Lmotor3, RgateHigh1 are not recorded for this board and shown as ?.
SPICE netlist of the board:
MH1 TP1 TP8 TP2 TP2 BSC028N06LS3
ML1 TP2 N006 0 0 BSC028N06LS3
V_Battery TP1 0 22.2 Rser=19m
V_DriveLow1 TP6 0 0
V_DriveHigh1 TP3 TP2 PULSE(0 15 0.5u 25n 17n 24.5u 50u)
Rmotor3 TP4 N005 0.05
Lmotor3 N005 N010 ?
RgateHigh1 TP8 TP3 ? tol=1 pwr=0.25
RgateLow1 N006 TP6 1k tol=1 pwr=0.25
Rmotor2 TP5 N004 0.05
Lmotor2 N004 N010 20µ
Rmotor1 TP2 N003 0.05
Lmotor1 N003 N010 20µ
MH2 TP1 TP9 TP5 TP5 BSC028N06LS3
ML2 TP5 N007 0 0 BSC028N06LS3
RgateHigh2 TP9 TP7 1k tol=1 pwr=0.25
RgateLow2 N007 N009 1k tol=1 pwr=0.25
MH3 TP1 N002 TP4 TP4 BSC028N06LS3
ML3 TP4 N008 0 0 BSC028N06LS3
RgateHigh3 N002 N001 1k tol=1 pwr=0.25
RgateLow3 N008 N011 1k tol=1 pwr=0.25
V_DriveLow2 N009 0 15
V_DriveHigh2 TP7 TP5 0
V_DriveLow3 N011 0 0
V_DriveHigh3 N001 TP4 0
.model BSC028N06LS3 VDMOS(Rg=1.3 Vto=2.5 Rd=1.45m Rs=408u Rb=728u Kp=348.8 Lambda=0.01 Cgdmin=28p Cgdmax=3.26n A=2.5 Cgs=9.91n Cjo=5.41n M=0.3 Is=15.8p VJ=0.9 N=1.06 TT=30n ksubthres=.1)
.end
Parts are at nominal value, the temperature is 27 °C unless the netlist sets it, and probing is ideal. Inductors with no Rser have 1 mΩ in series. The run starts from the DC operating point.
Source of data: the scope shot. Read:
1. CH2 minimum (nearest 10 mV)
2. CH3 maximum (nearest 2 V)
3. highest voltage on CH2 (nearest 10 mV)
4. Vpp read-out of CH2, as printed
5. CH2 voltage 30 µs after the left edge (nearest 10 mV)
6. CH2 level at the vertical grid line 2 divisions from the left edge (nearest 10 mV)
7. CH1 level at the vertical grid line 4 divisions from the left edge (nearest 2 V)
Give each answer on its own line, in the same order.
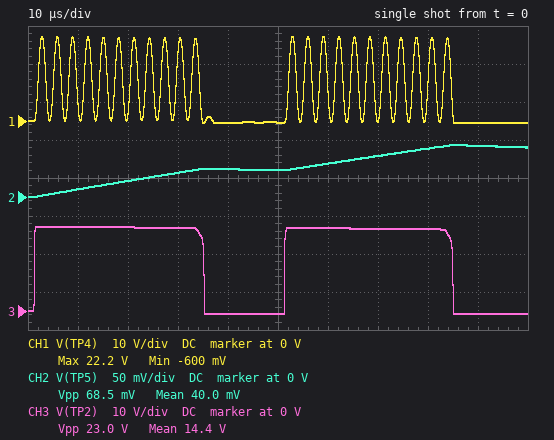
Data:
0 V
22 V
70 mV
68.5 mV
30 mV
20 mV
0 V
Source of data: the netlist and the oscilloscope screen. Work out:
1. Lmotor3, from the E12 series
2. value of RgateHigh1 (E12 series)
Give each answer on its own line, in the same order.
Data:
33 µH
390 Ω
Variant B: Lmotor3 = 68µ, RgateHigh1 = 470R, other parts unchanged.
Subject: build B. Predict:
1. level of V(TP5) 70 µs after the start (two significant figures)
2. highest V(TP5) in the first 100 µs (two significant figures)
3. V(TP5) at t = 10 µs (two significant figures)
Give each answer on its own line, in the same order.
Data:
56 mV
72 mV
9.8 mV
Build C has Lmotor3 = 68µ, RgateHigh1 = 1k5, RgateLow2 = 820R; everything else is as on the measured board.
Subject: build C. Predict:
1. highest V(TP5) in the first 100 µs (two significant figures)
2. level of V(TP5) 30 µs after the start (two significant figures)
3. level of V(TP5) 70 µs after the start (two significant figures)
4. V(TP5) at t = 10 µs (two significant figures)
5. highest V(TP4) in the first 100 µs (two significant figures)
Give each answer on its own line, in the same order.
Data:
97 mV
30 mV
70 mV
7.7 mV
22 V
